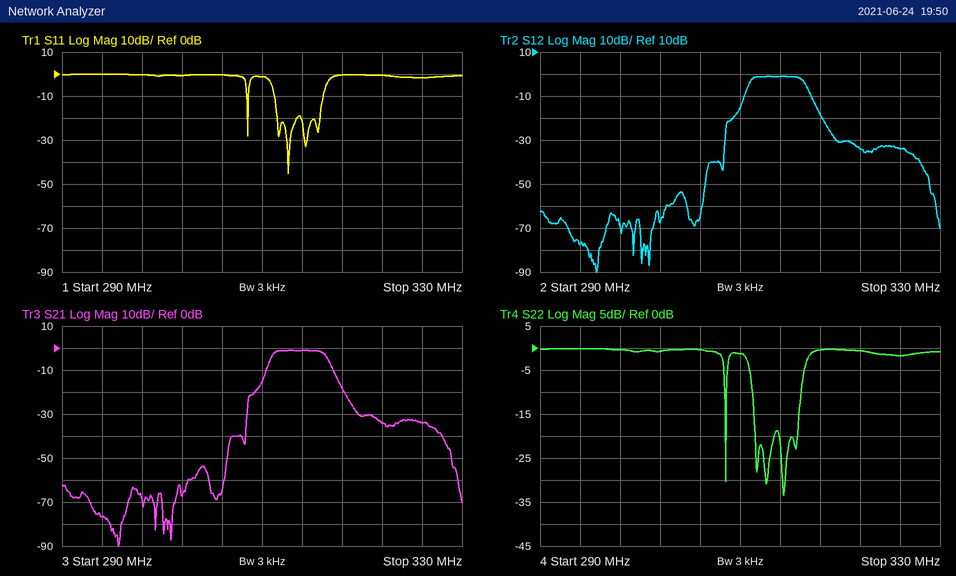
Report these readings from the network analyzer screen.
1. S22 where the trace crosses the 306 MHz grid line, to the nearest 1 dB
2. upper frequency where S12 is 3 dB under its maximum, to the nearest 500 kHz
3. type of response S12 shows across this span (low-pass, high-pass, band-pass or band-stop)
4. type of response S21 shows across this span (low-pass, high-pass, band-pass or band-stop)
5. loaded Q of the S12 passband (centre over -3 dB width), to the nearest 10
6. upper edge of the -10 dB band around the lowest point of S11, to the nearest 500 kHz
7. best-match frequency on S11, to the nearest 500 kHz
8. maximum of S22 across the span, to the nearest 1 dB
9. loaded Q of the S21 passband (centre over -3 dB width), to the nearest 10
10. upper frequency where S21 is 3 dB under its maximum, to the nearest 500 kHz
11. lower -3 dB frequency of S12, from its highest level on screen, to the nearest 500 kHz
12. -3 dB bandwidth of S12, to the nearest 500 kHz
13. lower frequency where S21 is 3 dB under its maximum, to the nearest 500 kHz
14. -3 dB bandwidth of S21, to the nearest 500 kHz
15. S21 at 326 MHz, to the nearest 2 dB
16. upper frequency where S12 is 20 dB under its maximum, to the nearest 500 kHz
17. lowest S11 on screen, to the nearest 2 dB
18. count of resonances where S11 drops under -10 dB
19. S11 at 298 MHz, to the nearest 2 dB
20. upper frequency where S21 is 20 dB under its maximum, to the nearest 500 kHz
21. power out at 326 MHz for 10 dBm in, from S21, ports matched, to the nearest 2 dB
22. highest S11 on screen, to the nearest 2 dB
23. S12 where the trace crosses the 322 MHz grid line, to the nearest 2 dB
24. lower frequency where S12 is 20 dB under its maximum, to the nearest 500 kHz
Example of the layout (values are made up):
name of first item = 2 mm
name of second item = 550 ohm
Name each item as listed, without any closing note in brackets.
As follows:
S22 where the trace crosses the 306 MHz grid line, to the nearest 1 dB = 0 dB
upper frequency where S12 is 3 dB under its maximum, to the nearest 500 kHz = 316.5 MHz
type of response S12 shows across this span = band-pass
type of response S21 shows across this span = band-pass
loaded Q of the S12 passband (centre over -3 dB width), to the nearest 10 = 60
upper edge of the -10 dB band around the lowest point of S11, to the nearest 500 kHz = 316.0 MHz
best-match frequency on S11, to the nearest 500 kHz = 312.5 MHz
maximum of S22 across the span, to the nearest 1 dB = 0 dB
loaded Q of the S21 passband (centre over -3 dB width), to the nearest 10 = 60
upper frequency where S21 is 3 dB under its maximum, to the nearest 500 kHz = 316.5 MHz
lower -3 dB frequency of S12, from its highest level on screen, to the nearest 500 kHz = 311.0 MHz
-3 dB bandwidth of S12, to the nearest 500 kHz = 5.5 MHz
lower frequency where S21 is 3 dB under its maximum, to the nearest 500 kHz = 311.0 MHz
-3 dB bandwidth of S21, to the nearest 500 kHz = 5.5 MHz
S21 at 326 MHz, to the nearest 2 dB = -34 dB
upper frequency where S12 is 20 dB under its maximum, to the nearest 500 kHz = 318.5 MHz
lowest S11 on screen, to the nearest 2 dB = -46 dB
count of resonances where S11 drops under -10 dB = 5
S11 at 298 MHz, to the nearest 2 dB = 0 dB
upper frequency where S21 is 20 dB under its maximum, to the nearest 500 kHz = 318.5 MHz
power out at 326 MHz for 10 dBm in, from S21, ports matched, to the nearest 2 dB = -24 dBm
highest S11 on screen, to the nearest 2 dB = 0 dB
S12 where the trace crosses the 322 MHz grid line, to the nearest 2 dB = -34 dB
lower frequency where S12 is 20 dB under its maximum, to the nearest 500 kHz = 309.0 MHz
